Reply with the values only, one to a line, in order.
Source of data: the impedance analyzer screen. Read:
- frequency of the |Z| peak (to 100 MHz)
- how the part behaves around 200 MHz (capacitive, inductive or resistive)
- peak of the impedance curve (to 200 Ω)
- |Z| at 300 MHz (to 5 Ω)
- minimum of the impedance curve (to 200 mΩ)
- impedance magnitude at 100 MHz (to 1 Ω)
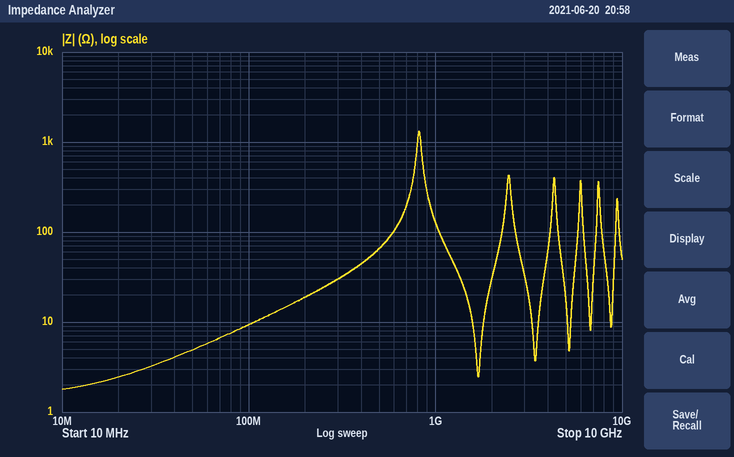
800 MHz
inductive
1.4 kΩ
30 Ω
1.8 Ω
9 Ω
